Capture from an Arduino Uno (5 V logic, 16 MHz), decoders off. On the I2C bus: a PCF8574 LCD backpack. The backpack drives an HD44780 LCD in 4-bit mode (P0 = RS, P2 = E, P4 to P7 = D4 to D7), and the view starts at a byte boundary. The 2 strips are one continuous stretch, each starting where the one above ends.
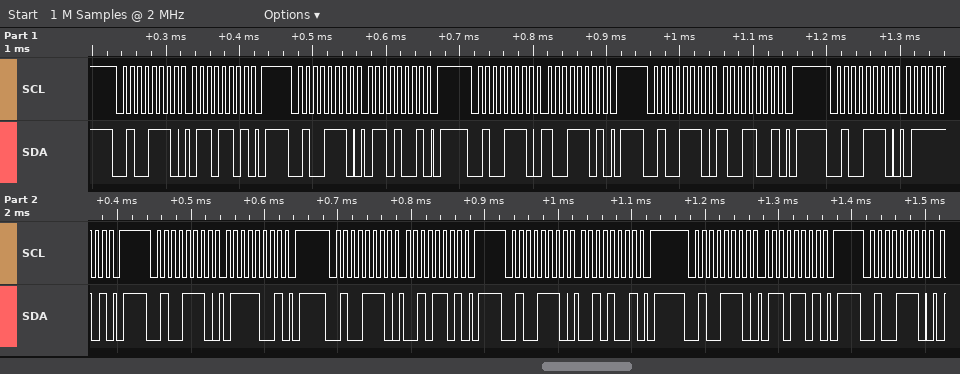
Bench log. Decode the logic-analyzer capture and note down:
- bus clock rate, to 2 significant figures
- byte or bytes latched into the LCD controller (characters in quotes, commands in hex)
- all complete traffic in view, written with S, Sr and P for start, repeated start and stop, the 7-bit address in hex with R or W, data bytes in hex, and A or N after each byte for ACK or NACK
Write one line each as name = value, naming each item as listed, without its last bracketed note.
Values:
bus clock rate, to 2 significant figures = 100 kHz
byte or bytes latched into the LCD controller = 'i' 'r'
all complete traffic in view, written with S, Sr and P for start, repeated start and stop, the 7-bit address in hex with R or W, data bytes in hex, and A or N after each byte for ACK or NACK = S 27W A 6D A P S 27W A 69 A P S 27W A 9D A P S 27W A 99 A P S 27W A 7D A P S 27W A 79 A P S 27W A 2D A P S 27W A 29 A P S 27W A 6D A P S 27W A
